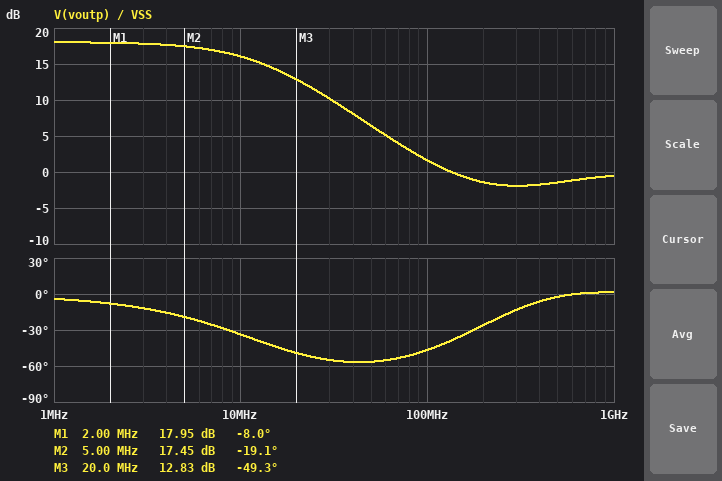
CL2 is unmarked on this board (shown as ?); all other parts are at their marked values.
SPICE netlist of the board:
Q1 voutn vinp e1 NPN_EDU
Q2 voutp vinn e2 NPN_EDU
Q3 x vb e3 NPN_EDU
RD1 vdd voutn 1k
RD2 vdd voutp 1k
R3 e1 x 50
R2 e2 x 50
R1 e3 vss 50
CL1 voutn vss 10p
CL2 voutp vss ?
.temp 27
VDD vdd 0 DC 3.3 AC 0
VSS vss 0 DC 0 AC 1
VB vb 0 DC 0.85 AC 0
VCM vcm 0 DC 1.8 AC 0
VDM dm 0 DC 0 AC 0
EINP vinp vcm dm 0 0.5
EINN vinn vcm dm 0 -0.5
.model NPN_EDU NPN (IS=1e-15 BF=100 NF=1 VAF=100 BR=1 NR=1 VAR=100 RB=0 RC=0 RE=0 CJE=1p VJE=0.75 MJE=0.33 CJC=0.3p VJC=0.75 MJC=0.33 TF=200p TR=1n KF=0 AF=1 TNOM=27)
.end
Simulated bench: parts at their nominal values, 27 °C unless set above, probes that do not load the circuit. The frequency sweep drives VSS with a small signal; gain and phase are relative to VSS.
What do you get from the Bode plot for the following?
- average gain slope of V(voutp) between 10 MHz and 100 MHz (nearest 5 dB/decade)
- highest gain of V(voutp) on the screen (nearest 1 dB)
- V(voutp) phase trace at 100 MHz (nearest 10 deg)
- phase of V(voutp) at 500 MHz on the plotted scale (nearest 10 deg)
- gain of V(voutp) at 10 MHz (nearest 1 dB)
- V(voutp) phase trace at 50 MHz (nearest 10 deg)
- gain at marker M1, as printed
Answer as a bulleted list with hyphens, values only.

- -15 dB/decade
- 18 dB
- -50 deg
- 0 deg
- 16 dB
- -60 deg
- 17.95 dB
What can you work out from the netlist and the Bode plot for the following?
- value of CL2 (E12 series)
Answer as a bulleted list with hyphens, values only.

- 12 pF
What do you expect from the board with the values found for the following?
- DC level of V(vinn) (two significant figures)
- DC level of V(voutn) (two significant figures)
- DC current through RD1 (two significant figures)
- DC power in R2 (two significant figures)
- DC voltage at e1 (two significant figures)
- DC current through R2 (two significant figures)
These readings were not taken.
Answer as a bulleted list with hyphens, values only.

- 1.8 V
- 2.2 V
- 1.1 mA
- 64 µW
- 1.1 V
- 1.1 mA
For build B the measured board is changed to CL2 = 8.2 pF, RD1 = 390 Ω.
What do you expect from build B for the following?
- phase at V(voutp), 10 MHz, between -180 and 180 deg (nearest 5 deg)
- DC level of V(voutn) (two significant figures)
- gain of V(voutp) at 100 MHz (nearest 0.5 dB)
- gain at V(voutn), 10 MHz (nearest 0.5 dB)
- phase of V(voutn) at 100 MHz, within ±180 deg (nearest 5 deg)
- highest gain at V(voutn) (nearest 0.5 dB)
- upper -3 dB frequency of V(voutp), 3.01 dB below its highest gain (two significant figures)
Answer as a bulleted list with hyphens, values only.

- -25 deg
- 2.9 V
- 3.5 dB
- 9.5 dB
- -40 deg
- 10.0 dB
- 19 MHz
